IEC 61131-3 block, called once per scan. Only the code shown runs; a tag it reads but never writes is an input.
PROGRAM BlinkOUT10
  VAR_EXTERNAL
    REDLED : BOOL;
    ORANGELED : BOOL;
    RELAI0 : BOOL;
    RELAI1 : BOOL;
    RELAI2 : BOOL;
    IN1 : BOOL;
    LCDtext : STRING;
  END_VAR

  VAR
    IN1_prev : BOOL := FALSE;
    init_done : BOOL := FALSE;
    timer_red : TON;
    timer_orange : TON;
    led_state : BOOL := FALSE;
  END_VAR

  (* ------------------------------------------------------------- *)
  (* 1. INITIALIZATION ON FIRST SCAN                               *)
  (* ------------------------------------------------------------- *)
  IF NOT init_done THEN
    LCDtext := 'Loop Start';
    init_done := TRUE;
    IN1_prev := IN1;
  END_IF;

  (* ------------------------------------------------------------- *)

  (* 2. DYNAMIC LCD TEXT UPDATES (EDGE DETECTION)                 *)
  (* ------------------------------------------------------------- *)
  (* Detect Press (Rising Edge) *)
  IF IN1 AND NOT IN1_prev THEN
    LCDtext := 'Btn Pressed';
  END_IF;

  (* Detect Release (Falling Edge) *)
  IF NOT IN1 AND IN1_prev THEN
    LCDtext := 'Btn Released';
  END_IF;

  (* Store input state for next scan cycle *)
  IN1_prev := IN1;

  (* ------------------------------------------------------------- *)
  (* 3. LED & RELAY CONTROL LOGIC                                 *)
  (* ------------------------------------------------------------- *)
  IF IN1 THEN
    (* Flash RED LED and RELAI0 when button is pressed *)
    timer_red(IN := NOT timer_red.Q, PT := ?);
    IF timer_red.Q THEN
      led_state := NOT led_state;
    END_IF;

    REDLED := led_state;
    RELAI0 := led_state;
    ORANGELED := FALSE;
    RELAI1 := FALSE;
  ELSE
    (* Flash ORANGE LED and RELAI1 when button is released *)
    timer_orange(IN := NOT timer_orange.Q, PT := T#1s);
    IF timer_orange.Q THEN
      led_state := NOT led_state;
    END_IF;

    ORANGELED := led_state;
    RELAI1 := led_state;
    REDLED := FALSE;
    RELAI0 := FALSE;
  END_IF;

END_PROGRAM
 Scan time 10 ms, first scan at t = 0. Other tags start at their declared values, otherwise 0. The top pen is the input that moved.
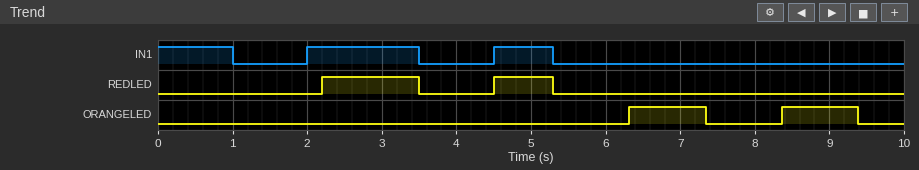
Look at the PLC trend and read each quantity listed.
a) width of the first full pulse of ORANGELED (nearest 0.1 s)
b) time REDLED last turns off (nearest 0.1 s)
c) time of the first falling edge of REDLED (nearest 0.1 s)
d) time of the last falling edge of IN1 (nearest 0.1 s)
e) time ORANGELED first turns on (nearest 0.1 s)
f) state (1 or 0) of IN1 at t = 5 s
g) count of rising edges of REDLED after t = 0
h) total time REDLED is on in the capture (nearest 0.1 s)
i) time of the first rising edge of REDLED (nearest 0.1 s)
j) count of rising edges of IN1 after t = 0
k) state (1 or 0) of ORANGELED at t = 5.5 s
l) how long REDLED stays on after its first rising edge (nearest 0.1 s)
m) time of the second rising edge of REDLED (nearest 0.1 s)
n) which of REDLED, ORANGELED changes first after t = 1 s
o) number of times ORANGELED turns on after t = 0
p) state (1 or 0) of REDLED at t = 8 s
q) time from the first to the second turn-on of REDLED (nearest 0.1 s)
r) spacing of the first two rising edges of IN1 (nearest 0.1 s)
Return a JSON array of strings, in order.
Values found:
["1.0 s", "5.3 s", "3.5 s", "5.3 s", "6.3 s", "1", "2", "2.1 s", "2.2 s", "2", "0", "1.3 s", "4.5 s", "REDLED", "2", "0", "2.3 s", "2.5 s"]
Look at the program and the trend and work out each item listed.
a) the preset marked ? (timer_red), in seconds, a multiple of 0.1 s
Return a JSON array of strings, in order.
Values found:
["2.2 s"]
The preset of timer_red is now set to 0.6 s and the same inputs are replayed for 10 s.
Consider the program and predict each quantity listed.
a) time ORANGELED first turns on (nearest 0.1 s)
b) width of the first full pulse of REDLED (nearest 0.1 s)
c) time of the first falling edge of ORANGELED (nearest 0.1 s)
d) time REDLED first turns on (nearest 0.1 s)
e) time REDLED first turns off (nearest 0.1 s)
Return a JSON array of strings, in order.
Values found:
["1.0 s", "0.4 s", "2.0 s", "0.6 s", "1.0 s"]
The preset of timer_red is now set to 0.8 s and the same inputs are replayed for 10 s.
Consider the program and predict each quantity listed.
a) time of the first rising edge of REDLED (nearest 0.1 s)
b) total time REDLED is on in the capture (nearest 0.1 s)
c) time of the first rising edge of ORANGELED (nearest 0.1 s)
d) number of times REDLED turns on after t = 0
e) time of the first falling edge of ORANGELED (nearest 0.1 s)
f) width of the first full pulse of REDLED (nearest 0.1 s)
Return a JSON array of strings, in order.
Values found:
["0.8 s", "1.7 s", "1.0 s", "3", "2.0 s", "0.2 s"]
